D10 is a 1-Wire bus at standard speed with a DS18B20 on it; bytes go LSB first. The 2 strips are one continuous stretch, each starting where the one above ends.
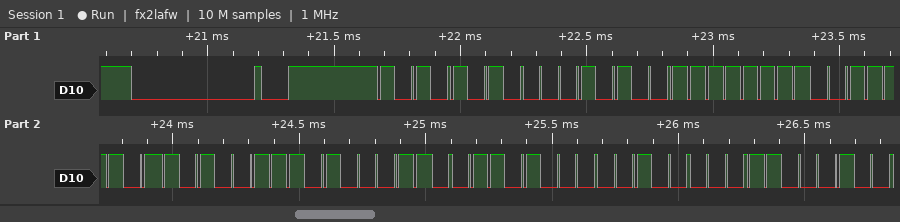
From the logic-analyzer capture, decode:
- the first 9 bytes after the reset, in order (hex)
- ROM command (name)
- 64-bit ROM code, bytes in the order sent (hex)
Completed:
55 28 FF BC E5 62 16 04 23
Match ROM
28 FF BC E5 62 16 04 23
